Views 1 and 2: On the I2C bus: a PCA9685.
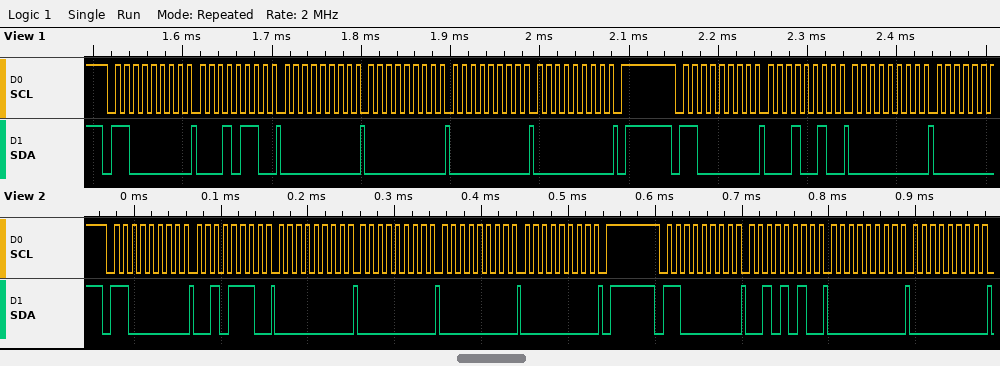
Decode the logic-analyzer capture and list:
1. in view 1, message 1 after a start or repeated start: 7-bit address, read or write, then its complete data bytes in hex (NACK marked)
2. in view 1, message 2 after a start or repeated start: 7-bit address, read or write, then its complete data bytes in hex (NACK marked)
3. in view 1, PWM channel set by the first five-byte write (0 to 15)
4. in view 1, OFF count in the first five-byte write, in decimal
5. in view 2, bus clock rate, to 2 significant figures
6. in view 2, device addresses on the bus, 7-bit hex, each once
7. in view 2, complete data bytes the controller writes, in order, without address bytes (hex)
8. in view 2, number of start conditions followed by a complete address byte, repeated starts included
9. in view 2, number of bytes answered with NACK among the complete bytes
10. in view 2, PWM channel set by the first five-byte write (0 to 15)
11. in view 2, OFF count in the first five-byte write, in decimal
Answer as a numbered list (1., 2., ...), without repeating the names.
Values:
1. 0x60 write: 16 00 00 00 00
2. 0x60 write: 12 00
3. 4
4. 0
5. 100 kHz
6. 0x60
7. 2E 00 00 00 00 2A 00 00
8. 2
9. 0
10. 10
11. 0
